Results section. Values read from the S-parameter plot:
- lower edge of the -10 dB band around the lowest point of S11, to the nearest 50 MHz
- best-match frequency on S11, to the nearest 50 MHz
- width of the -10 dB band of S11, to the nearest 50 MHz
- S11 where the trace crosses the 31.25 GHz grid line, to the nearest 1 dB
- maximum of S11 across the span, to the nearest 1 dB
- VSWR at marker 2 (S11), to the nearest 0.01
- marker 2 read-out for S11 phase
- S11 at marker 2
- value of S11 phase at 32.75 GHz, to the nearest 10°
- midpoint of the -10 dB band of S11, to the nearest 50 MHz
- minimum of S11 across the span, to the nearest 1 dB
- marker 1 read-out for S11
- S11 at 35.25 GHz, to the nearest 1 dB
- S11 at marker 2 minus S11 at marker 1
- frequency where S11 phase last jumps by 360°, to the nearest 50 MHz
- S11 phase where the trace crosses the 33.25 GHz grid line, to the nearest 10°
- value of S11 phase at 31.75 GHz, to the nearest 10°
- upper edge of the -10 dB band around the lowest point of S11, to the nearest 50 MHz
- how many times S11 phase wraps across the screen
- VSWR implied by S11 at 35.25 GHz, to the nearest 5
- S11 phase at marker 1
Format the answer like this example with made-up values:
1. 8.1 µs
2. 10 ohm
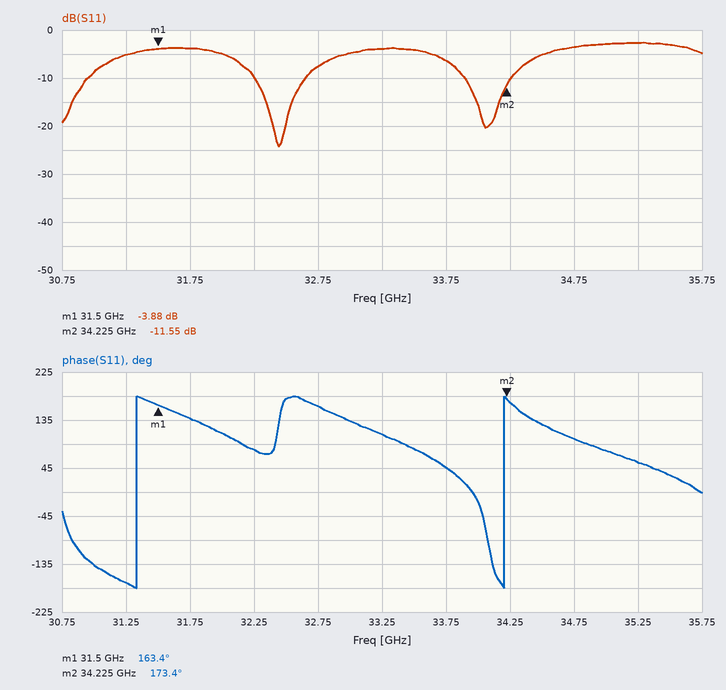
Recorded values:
1. 32.25 GHz
2. 32.45 GHz
3. 400 MHz
4. -5 dB
5. -3 dB
6. 1.72
7. 173.4°
8. -11.55 dB
9. 160°
10. 32.45 GHz
11. -24 dB
12. -3.88 dB
13. -3 dB
14. -7.67 dB
15. 34.20 GHz
16. 110°
17. 140°
18. 32.65 GHz
19. 2
20. 5
21. 163.4°
